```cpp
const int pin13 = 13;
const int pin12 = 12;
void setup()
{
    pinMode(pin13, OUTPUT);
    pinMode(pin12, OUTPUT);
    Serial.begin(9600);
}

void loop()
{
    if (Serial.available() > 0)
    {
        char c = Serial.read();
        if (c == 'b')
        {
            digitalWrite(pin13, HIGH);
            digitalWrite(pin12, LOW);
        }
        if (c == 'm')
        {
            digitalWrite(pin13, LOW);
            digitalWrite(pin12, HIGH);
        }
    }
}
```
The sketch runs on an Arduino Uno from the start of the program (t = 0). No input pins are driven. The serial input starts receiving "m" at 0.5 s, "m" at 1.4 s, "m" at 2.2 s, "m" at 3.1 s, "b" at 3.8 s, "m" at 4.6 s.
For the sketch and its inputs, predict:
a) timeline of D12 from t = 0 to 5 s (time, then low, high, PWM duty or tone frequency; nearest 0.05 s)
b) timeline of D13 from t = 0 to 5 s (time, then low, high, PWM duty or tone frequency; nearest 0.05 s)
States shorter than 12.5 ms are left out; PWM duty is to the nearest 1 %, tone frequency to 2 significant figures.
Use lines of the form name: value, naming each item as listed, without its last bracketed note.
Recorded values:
timeline of D12 from t = 0 to 5 s: 0 s low; 0.5 s high; 3.8 s low; 4.6 s high
timeline of D13 from t = 0 to 5 s: 0 s low; 3.8 s high; 4.6 s low
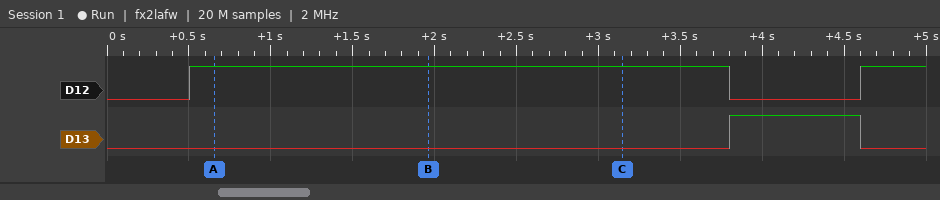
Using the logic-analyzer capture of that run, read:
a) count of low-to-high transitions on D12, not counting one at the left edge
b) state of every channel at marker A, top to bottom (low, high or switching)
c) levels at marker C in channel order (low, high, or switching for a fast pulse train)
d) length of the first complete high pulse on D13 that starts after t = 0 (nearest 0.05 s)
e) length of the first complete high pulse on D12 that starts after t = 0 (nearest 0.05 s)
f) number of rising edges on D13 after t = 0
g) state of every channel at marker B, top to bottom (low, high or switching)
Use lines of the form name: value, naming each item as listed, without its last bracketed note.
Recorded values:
count of low-to-high transitions on D12, not counting one at the left edge: 2
state of every channel at marker A, top to bottom: D12 high, D13 low
levels at marker C in channel order: D12 high, D13 low
length of the first complete high pulse on D13 that starts after t = 0: 0.80 s
length of the first complete high pulse on D12 that starts after t = 0: 3.30 s
number of rising edges on D13 after t = 0: 1
state of every channel at marker B, top to bottom: D12 high, D13 low
